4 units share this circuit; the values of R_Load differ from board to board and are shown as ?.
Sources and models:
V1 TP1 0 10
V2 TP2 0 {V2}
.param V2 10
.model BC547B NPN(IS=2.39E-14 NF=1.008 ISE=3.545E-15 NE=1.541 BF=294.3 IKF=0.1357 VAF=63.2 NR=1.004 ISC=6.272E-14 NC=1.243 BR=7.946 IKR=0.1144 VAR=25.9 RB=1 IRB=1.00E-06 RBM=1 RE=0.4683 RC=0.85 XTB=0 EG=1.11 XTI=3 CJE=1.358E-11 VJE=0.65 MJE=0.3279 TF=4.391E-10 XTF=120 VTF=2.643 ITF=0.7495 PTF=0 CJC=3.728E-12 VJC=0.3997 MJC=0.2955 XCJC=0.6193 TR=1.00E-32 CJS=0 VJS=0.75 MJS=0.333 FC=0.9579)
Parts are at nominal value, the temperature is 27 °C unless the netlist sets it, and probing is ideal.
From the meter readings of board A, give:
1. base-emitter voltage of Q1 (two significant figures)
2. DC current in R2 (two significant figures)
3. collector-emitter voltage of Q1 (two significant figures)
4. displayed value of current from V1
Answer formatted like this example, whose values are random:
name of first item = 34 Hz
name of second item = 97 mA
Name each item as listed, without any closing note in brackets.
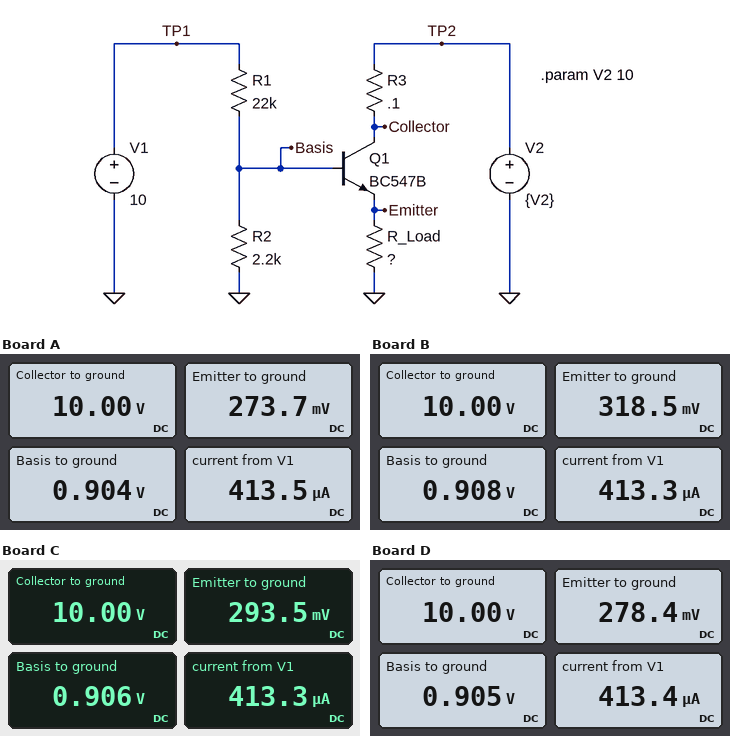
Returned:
base-emitter voltage of Q1 = 630 mV
DC current in R2 = 410 µA
collector-emitter voltage of Q1 = 9.7 V
displayed value of current from V1 = 413.5 µA
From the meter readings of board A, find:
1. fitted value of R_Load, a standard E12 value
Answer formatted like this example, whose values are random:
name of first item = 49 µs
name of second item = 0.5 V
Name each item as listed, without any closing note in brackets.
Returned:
fitted value of R_Load, a standard E12 value = 330 Ω
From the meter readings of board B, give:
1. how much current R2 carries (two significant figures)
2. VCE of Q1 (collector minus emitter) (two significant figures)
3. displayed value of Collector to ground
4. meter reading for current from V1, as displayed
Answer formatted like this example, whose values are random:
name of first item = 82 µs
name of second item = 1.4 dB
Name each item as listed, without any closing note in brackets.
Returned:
how much current R2 carries = 410 µA
VCE of Q1 (collector minus emitter) = 9.7 V
displayed value of Collector to ground = 10.00 V
meter reading for current from V1, as displayed = 413.3 µA
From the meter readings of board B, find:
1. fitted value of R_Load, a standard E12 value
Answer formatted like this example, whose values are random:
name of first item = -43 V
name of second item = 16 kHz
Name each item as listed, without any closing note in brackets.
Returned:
fitted value of R_Load, a standard E12 value = 1.8 kΩ
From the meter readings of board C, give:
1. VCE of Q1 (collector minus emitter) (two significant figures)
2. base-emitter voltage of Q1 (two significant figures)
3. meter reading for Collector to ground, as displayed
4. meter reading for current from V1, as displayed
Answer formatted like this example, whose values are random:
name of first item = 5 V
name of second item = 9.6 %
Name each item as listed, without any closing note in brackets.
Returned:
VCE of Q1 (collector minus emitter) = 9.7 V
base-emitter voltage of Q1 = 610 mV
meter reading for Collector to ground, as displayed = 10.00 V
meter reading for current from V1, as displayed = 413.3 µA
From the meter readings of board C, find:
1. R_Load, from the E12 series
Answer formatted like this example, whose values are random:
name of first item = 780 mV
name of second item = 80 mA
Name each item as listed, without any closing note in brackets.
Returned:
R_Load, from the E12 series = 680 Ω
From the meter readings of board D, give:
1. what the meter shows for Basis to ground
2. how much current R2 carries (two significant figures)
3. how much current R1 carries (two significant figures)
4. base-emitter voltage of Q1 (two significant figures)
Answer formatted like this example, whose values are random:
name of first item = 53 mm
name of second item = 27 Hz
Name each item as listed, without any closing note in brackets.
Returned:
what the meter shows for Basis to ground = 0.905 V
how much current R2 carries = 410 µA
how much current R1 carries = 410 µA
base-emitter voltage of Q1 = 630 mV
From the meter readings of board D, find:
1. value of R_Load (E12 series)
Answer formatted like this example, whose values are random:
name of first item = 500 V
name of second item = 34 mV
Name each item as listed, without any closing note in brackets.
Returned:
value of R_Load = 390 Ω
